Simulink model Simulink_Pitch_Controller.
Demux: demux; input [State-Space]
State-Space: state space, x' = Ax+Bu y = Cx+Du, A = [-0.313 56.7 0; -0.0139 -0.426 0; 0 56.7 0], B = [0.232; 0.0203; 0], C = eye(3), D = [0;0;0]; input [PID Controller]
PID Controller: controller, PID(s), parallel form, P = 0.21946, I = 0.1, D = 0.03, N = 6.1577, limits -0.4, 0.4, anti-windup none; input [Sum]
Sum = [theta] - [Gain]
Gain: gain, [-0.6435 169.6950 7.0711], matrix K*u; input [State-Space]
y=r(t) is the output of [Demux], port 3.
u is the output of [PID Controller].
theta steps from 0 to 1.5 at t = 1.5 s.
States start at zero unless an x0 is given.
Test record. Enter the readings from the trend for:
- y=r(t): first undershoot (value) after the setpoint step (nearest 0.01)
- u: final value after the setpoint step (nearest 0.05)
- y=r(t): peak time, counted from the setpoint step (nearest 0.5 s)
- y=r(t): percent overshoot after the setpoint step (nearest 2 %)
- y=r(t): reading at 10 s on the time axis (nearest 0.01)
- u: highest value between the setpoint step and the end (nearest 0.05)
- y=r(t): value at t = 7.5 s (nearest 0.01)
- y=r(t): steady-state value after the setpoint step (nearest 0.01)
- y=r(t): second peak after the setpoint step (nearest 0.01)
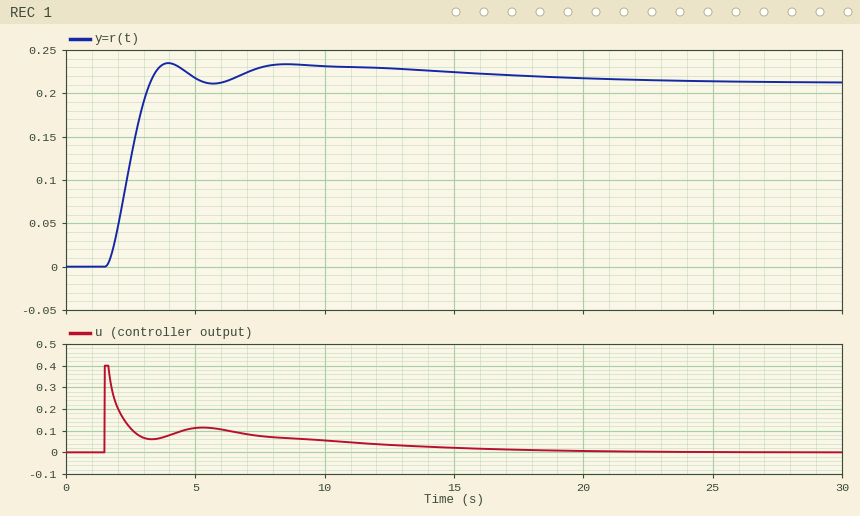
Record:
0.21
0.00
2.5 s
10 %
0.23
0.40
0.23
0.21
0.23
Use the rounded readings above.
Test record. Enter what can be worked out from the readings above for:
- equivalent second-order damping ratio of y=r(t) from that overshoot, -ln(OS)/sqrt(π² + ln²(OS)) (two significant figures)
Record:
0.59
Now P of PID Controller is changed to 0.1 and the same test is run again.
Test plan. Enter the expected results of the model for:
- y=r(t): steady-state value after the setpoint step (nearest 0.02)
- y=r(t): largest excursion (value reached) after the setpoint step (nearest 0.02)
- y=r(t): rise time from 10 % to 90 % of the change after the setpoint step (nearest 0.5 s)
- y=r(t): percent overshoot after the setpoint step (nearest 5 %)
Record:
0.22
0.24
1.5 s
15 %
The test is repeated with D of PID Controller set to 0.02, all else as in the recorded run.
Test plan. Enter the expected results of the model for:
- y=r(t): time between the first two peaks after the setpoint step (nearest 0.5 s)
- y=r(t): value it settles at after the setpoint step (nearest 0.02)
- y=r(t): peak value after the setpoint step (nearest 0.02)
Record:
4.5 s
0.22
0.24
